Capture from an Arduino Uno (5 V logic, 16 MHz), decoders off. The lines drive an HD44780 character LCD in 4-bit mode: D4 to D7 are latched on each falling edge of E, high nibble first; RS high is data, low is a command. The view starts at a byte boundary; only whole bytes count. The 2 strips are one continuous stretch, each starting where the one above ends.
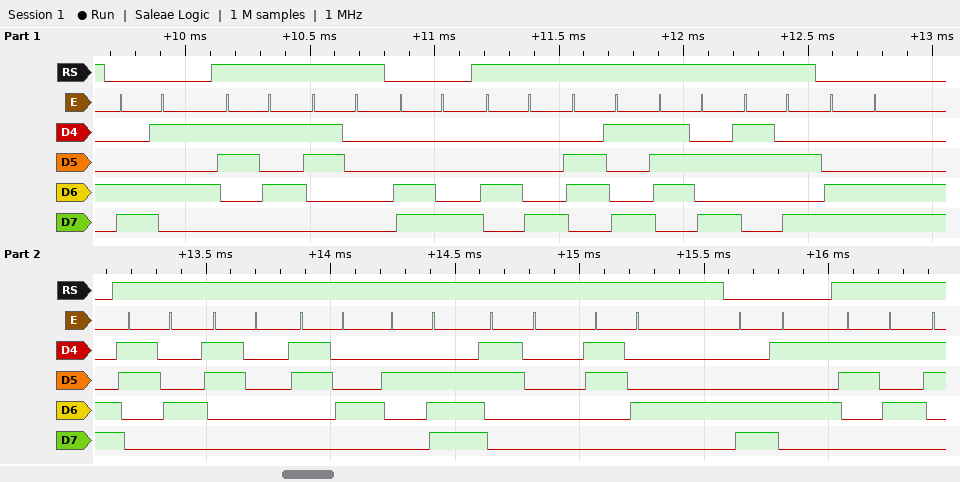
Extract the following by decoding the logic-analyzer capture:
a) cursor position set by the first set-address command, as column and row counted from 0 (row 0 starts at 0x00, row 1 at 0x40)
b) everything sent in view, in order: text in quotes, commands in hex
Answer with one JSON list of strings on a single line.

["column 5, row 1", "0xC5 \"50\" 0xC8 \"Hiz:\" 0xCC \"404.04\" 0xC5 \"5\""]
